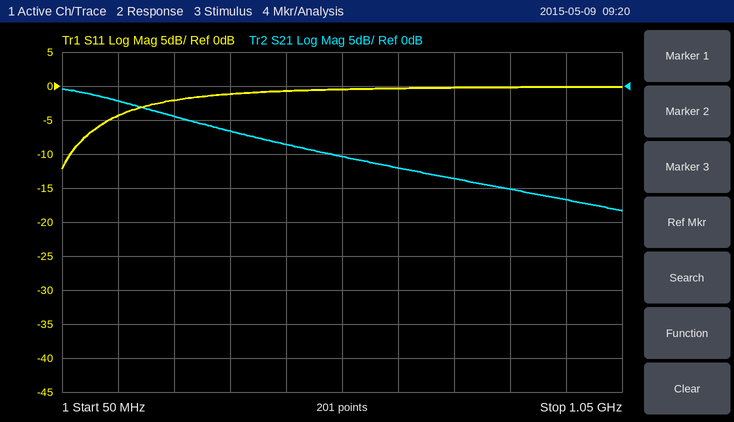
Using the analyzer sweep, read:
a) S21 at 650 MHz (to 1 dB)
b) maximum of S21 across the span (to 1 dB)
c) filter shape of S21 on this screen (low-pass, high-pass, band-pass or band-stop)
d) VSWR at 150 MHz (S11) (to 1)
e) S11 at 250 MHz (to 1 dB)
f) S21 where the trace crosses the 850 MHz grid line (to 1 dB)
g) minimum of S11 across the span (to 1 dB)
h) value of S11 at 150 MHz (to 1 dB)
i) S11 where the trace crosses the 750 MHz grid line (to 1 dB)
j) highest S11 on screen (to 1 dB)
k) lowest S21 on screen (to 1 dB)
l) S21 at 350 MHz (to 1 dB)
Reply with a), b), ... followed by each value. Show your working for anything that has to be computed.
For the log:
a) -12 dB
b) 0 dB
c) low-pass
d) |Γ| = 10^(-4/20) = 0.6310; VSWR = (1 + 0.6310)/(1 − 0.6310) ≈ 4
e) -2 dB
f) -15 dB
g) -12 dB
h) -4 dB
i) 0 dB
j) 0 dB
k) -18 dB
l) -7 dB
